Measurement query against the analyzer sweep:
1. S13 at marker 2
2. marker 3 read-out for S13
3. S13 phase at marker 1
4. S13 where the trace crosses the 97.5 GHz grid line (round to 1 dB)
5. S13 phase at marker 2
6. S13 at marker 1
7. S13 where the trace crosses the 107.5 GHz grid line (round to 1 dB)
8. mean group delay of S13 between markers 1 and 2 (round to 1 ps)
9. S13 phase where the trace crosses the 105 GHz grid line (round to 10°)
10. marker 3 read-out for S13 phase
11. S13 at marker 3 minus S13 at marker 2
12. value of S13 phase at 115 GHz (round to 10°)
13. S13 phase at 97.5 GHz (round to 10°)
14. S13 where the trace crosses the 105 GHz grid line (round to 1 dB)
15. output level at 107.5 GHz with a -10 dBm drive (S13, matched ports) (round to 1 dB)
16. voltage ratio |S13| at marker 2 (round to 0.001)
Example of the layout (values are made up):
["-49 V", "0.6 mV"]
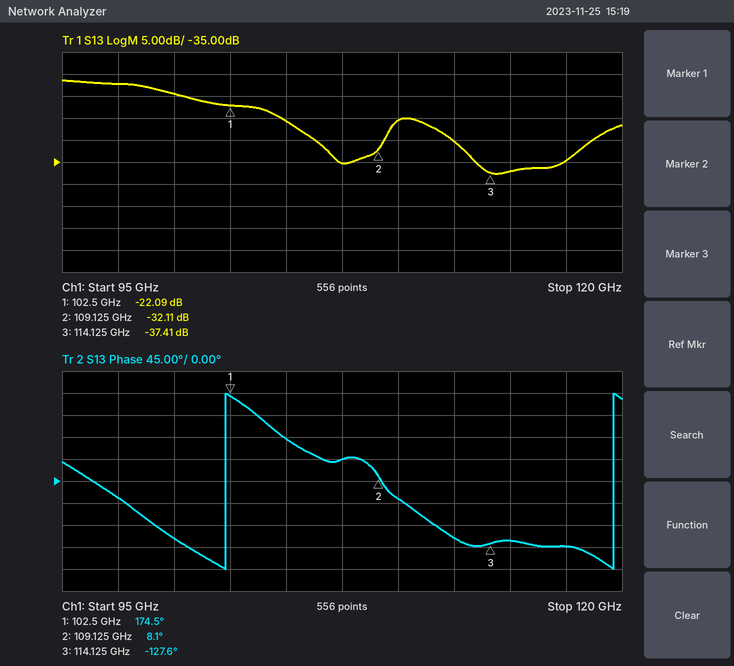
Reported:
["-32.11 dB", "-37.41 dB", "174.5°", "-17 dB", "8.1°", "-22.09 dB", "-35 dB", "70 ps", "90°", "-127.6°", "-5.30 dB", "-120°", "-30°", "-26 dB", "-45 dBm", "0.025"]
